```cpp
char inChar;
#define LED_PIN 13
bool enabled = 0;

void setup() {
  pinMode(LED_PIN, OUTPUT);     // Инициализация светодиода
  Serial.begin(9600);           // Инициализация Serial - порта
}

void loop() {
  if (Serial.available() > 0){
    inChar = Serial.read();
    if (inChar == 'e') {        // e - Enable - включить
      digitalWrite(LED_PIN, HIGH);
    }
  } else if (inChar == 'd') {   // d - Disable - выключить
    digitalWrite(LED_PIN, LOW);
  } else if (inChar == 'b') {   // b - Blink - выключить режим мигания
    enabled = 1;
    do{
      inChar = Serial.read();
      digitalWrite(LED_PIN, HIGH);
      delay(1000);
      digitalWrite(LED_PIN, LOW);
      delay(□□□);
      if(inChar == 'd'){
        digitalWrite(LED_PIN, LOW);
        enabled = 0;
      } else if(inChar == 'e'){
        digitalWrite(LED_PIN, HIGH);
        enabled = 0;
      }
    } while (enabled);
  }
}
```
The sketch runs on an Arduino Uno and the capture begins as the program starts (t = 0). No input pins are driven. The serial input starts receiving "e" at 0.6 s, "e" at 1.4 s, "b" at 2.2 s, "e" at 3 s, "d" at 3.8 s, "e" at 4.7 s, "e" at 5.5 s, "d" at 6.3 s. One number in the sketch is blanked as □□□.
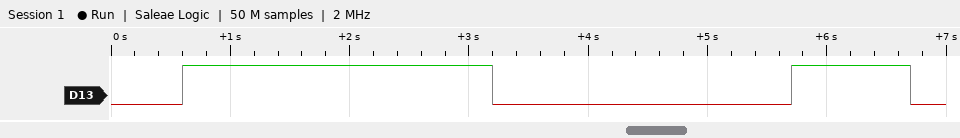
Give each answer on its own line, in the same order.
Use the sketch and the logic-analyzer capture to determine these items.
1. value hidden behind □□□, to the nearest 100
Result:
2500
